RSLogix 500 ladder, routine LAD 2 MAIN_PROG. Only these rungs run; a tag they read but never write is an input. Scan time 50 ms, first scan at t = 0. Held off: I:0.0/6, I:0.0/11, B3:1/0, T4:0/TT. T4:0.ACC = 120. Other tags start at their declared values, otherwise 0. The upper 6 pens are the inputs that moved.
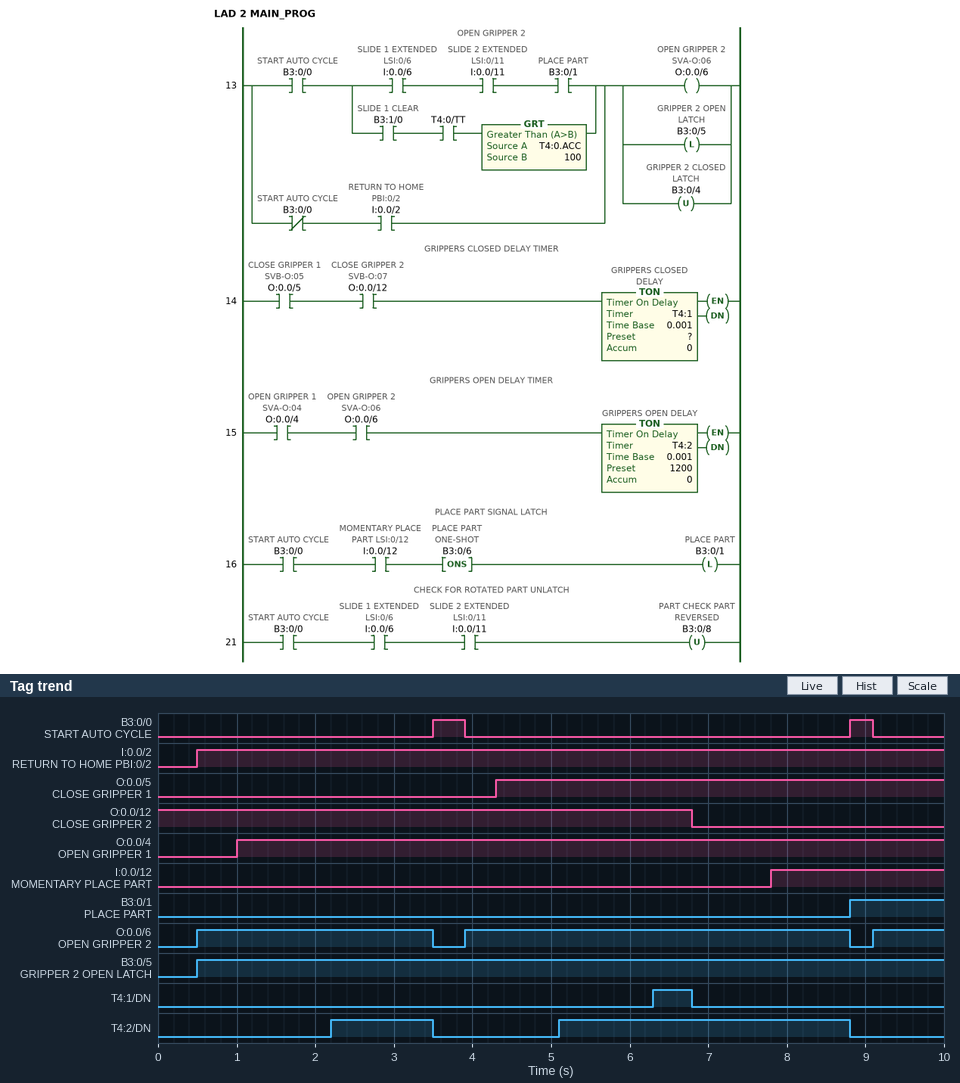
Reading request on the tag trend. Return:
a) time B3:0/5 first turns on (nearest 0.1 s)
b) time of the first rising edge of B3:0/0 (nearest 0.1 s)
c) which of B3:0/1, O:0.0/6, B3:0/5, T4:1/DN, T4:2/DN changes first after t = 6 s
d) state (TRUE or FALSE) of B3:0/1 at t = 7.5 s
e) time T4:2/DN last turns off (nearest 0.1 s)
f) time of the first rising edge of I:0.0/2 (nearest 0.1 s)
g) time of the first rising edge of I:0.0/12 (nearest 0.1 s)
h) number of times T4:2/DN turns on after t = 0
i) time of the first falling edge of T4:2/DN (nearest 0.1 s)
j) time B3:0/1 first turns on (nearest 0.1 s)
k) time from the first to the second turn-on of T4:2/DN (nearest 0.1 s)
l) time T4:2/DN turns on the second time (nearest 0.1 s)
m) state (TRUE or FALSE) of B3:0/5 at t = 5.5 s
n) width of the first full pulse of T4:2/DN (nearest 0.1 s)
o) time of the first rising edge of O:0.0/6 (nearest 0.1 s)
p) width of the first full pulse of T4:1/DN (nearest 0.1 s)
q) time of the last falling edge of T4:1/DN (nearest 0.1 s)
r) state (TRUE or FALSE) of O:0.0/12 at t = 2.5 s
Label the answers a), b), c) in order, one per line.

a) 0.5 s
b) 3.5 s
c) T4:1/DN
d) FALSE
e) 8.8 s
f) 0.5 s
g) 7.8 s
h) 2
i) 3.5 s
j) 8.8 s
k) 2.9 s
l) 5.1 s
m) TRUE
n) 1.3 s
o) 0.5 s
p) 0.5 s
q) 6.8 s
r) TRUE
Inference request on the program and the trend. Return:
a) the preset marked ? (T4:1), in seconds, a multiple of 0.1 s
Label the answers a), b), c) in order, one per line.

a) 2.0 s
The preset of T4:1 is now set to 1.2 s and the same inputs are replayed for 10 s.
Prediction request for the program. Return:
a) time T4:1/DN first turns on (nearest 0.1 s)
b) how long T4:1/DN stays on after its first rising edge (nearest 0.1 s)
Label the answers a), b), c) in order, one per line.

a) 5.5 s
b) 1.3 s
